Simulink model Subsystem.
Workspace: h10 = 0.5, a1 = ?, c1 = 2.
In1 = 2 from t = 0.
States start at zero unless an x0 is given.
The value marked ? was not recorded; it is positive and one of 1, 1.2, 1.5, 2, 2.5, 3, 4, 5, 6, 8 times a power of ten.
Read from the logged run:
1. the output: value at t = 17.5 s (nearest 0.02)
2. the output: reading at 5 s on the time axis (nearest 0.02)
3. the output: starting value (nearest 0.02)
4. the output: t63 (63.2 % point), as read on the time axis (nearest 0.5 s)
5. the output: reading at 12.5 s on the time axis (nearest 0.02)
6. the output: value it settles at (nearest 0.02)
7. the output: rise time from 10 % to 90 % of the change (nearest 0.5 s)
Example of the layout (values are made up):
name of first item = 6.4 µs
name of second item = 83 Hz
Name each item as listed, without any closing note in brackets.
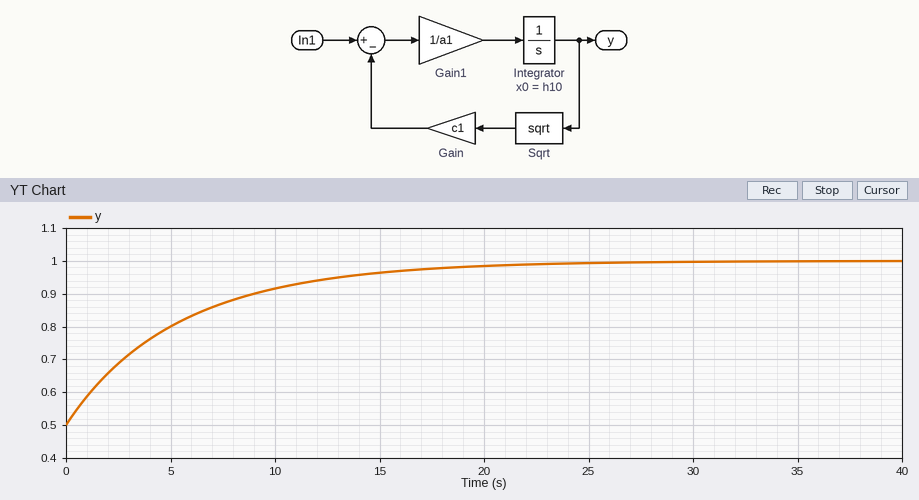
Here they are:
the output: value at t = 17.5 s = 0.98
the output: reading at 5 s on the time axis = 0.80
the output: starting value = 0.50
the output: t63 (63.2 % point), as read on the time axis = 5.5 s
the output: reading at 12.5 s on the time axis = 0.94
the output: value it settles at = 1.00
the output: rise time from 10 % to 90 % of the change = 12.5 s
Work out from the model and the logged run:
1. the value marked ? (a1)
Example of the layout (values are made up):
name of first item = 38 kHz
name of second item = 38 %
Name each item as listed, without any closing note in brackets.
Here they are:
the value marked ? = 6
